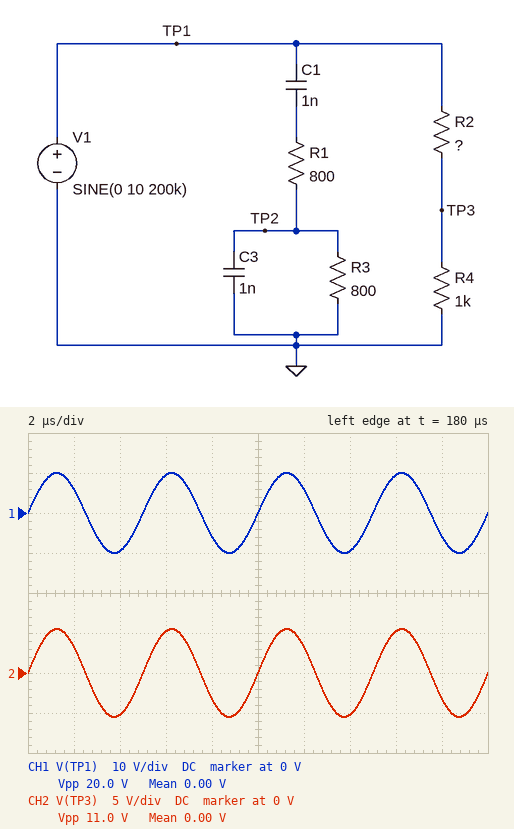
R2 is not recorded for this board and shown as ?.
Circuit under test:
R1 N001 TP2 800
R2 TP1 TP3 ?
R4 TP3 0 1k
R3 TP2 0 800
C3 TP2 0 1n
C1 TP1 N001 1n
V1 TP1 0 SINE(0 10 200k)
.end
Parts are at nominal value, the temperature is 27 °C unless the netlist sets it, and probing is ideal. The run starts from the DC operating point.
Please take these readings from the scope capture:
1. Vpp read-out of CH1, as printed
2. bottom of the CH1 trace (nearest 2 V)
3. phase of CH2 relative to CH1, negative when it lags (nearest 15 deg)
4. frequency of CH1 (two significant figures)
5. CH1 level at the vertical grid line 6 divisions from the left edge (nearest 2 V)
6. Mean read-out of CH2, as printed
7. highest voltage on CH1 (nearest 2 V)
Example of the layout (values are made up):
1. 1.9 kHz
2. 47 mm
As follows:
1. 20.0 V
2. -10 V
3. 0 deg
4. 200 kHz
5. 6 V
6. 0.00 V
7. 10 V
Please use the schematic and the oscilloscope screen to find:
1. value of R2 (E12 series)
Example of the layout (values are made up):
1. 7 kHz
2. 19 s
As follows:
1. 820 Ω
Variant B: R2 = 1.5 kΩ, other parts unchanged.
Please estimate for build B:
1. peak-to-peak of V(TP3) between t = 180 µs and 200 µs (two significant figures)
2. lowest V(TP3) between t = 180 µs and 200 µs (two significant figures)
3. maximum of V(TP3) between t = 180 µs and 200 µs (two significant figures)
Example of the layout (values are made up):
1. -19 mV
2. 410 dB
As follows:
1. 8.0 V
2. -4.0 V
3. 4.0 V
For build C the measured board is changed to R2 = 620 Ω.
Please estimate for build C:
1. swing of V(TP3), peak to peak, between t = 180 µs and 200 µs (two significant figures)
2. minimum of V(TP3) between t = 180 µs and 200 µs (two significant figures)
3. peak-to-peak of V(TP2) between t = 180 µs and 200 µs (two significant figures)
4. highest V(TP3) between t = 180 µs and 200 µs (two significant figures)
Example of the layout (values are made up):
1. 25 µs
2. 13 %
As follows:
1. 12 V
2. -6.2 V
3. 6.7 V
4. 6.2 V
